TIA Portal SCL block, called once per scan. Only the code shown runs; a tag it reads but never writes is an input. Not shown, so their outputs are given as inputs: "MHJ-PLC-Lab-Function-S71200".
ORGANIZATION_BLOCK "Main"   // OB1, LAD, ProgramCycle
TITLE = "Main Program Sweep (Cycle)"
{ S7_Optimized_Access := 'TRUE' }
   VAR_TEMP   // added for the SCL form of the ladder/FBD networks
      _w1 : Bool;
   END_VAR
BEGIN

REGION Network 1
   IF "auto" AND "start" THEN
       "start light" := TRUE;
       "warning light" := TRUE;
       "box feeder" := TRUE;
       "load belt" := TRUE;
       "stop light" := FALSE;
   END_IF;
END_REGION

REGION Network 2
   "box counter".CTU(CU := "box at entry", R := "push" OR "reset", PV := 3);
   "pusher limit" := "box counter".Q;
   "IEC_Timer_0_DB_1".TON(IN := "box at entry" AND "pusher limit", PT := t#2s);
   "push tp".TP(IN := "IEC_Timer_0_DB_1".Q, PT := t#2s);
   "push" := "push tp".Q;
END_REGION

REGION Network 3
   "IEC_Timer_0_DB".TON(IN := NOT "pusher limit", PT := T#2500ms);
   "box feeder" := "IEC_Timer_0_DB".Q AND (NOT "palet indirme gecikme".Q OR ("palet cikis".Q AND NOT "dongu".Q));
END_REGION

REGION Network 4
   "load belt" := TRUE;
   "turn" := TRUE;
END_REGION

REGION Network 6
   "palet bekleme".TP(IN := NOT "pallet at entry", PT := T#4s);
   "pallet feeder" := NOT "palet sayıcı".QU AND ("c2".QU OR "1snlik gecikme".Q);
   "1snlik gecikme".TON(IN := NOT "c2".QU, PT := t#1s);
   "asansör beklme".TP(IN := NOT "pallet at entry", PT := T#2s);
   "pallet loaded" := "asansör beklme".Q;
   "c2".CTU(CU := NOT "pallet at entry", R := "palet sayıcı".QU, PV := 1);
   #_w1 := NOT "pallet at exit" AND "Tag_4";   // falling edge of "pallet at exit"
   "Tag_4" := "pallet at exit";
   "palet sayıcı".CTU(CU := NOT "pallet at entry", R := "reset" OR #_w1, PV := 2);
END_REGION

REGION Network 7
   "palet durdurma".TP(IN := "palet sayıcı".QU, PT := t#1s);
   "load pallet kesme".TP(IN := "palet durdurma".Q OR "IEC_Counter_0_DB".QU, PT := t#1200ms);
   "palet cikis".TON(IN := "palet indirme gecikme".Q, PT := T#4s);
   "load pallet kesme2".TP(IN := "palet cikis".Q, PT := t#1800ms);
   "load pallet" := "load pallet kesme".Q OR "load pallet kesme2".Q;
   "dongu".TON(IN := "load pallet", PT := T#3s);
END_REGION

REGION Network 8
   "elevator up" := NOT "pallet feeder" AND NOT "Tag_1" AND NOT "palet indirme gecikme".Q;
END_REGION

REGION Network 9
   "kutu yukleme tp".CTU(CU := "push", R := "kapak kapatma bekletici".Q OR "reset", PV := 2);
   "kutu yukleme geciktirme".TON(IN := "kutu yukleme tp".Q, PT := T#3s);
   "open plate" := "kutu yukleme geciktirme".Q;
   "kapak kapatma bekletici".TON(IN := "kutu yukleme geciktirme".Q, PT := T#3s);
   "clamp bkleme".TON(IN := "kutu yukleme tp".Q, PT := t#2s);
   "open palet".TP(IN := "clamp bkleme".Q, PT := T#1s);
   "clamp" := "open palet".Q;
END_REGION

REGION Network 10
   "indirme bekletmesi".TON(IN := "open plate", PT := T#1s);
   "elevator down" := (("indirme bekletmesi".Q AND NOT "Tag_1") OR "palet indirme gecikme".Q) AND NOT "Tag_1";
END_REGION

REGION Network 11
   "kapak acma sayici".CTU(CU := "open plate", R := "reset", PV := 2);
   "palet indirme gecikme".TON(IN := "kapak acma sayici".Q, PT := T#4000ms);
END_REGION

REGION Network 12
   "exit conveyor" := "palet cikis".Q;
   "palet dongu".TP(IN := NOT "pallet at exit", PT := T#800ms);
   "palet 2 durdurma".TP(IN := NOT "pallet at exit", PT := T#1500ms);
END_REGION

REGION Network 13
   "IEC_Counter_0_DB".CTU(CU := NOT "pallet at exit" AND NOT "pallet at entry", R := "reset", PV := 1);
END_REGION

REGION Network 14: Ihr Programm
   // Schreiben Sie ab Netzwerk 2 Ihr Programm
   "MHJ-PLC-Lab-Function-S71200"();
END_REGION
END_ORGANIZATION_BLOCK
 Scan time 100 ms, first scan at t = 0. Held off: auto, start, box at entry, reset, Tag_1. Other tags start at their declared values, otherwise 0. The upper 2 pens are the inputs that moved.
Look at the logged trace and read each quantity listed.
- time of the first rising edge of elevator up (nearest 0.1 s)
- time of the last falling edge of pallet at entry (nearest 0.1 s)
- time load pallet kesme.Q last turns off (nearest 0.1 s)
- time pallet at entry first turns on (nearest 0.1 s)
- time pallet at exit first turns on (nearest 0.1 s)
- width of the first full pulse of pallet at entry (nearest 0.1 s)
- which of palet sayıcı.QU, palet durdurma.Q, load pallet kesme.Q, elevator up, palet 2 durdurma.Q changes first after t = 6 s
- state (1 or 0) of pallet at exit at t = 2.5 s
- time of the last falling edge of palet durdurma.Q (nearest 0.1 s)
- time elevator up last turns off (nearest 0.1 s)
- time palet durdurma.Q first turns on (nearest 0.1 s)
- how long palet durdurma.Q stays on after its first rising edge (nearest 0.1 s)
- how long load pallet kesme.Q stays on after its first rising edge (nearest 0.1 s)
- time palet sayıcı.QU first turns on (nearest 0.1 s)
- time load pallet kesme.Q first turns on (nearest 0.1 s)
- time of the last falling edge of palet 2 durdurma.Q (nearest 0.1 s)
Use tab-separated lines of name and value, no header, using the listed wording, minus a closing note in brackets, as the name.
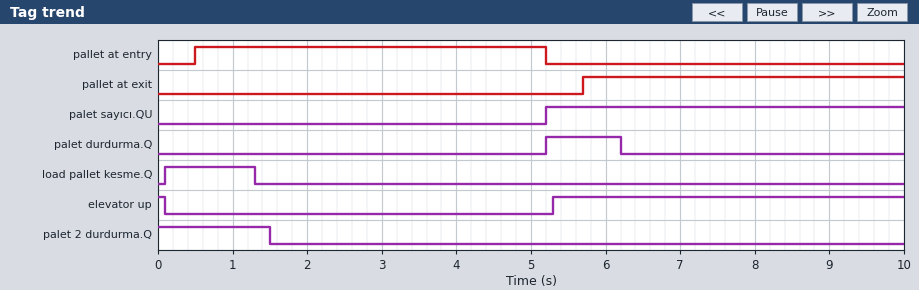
time of the first rising edge of elevator up	5.3 s
time of the last falling edge of pallet at entry	5.2 s
time load pallet kesme.Q last turns off	1.3 s
time pallet at entry first turns on	0.5 s
time pallet at exit first turns on	5.7 s
width of the first full pulse of pallet at entry	4.7 s
which of palet sayıcı.QU, palet durdurma.Q, load pallet kesme.Q, elevator up, palet 2 durdurma.Q changes first after t = 6 s	palet durdurma.Q
state (1 or 0) of pallet at exit at t = 2.5 s	0
time of the last falling edge of palet durdurma.Q	6.2 s
time elevator up last turns off	0.1 s
time palet durdurma.Q first turns on	5.2 s
how long palet durdurma.Q stays on after its first rising edge	1.0 s
how long load pallet kesme.Q stays on after its first rising edge	1.2 s
time palet sayıcı.QU first turns on	5.2 s
time load pallet kesme.Q first turns on	0.1 s
time of the last falling edge of palet 2 durdurma.Q	1.5 s
